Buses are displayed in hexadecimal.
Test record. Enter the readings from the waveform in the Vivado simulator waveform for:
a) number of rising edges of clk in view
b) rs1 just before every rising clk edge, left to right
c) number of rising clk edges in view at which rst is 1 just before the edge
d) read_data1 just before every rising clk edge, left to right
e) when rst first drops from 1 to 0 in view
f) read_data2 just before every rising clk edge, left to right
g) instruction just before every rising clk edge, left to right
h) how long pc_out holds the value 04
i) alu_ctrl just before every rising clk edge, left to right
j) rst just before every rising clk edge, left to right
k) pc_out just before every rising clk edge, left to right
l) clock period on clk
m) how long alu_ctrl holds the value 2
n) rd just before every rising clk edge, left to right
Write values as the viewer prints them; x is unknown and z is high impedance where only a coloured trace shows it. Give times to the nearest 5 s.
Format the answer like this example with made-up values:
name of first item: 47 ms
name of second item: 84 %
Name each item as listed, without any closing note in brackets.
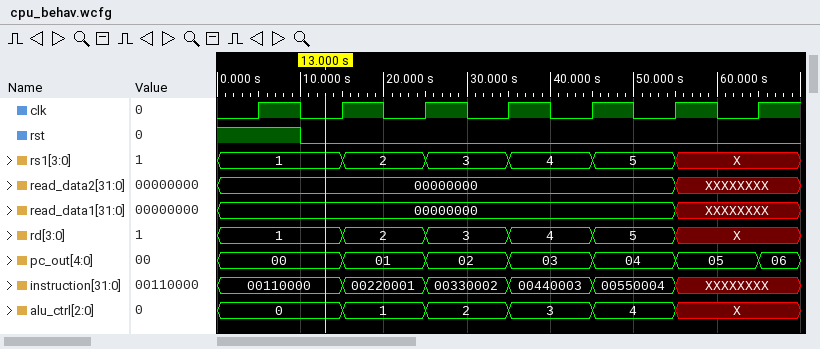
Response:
number of rising edges of clk in view: 7
rs1 just before every rising clk edge, left to right: 1, 1, 2, 3, 4, 5, X
number of rising clk edges in view at which rst is 1 just before the edge: 1
read_data1 just before every rising clk edge, left to right: 00000000, 00000000, 00000000, 00000000, 00000000, 00000000, XXXXXXXX
when rst first drops from 1 to 0 in view: 10 s
read_data2 just before every rising clk edge, left to right: 00000000, 00000000, 00000000, 00000000, 00000000, 00000000, XXXXXXXX
instruction just before every rising clk edge, left to right: 00110000, 00110000, 00220001, 00330002, 00440003, 00550004, XXXXXXXX
how long pc_out holds the value 04: 10 s
alu_ctrl just before every rising clk edge, left to right: 0, 0, 1, 2, 3, 4, X
rst just before every rising clk edge, left to right: 1 0 0 0 0 0 0
pc_out just before every rising clk edge, left to right: 00, 00, 01, 02, 03, 04, 05
clock period on clk: 10 s
how long alu_ctrl holds the value 2: 10 s
rd just before every rising clk edge, left to right: 1, 1, 2, 3, 4, 5, X
